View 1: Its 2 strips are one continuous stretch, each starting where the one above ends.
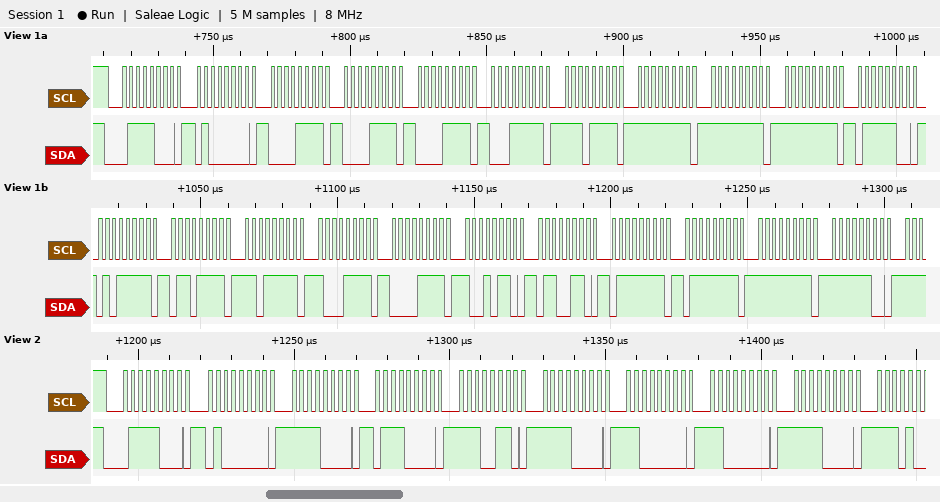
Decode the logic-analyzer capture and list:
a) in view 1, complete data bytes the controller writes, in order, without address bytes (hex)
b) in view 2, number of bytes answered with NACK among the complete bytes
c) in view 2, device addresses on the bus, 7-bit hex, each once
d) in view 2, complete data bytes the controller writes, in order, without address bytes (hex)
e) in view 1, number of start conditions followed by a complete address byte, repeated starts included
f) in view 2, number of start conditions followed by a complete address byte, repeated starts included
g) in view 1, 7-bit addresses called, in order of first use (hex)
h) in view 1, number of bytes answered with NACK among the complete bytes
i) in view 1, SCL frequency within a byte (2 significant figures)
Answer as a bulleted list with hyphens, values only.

- 40 0F 0F 0F 1F EF FF FF FF 7C 5F 6F DF 8F 0F 96 66 7F 7F FF FC
- 0
- 0x3C
- 40 F0 70 E6 F0 C0 C0 F0
- 1
- 1
- 0x3C
- 0
- 400 kHz
